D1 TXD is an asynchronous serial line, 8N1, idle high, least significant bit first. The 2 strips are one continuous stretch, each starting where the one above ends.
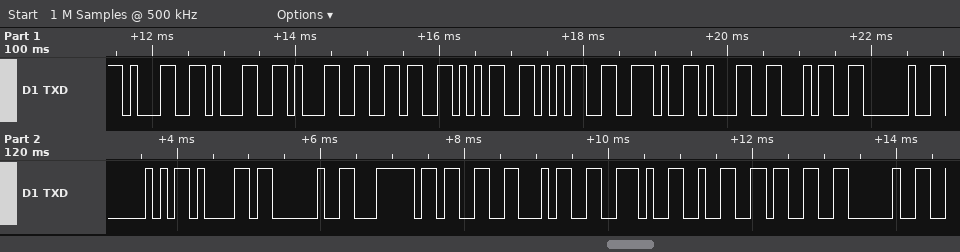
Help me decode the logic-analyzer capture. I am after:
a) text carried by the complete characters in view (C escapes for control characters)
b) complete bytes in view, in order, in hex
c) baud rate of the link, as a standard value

"111655.14 Pa |34.23 "
31 31 31 36 35 35 2E 31 34 20 50 61 20 7C 33 34 2E 32 33 20
9600 baud
